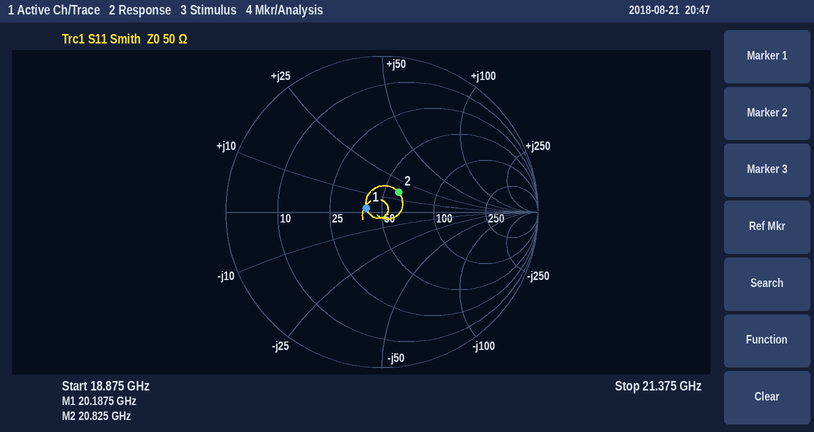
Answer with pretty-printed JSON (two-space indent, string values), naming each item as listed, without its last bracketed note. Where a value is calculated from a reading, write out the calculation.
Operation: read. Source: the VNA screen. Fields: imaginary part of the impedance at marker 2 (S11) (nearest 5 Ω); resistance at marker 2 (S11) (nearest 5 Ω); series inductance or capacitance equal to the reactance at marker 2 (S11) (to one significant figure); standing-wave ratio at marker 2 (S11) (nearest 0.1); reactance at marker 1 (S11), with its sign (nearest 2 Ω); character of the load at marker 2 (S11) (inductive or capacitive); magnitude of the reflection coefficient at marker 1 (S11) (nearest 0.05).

{
  "imaginary part of the impedance at marker 2 (S11)": "+15 Ω",
  "resistance at marker 2 (S11)": "60 Ω",
  "series inductance or capacitance equal to the reactance at marker 2 (S11)": "L = 15 Ω/(2π × 20.825 GHz) ≈ 115 pH, so 100 pH to one significant figure",
  "standing-wave ratio at marker 2 (S11)": "1.4",
  "reactance at marker 1 (S11), with its sign": "+2 Ω",
  "character of the load at marker 2 (S11)": "inductive",
  "magnitude of the reflection coefficient at marker 1 (S11)": "0.10"
}
